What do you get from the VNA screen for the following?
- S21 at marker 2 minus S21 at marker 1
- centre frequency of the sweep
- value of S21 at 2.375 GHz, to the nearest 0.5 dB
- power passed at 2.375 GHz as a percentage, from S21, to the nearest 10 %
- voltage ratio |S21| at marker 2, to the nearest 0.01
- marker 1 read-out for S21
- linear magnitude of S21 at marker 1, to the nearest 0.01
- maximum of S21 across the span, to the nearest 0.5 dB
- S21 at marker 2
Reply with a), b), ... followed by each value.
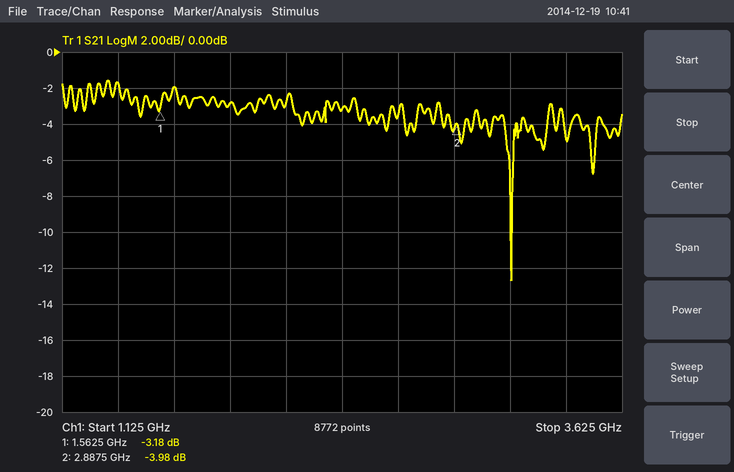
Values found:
a) -0.80 dB
b) 2.375 GHz
c) -3.0 dB
d) 50 %
e) 0.63
f) -3.18 dB
g) 0.69
h) -1.5 dB
i) -3.98 dB
